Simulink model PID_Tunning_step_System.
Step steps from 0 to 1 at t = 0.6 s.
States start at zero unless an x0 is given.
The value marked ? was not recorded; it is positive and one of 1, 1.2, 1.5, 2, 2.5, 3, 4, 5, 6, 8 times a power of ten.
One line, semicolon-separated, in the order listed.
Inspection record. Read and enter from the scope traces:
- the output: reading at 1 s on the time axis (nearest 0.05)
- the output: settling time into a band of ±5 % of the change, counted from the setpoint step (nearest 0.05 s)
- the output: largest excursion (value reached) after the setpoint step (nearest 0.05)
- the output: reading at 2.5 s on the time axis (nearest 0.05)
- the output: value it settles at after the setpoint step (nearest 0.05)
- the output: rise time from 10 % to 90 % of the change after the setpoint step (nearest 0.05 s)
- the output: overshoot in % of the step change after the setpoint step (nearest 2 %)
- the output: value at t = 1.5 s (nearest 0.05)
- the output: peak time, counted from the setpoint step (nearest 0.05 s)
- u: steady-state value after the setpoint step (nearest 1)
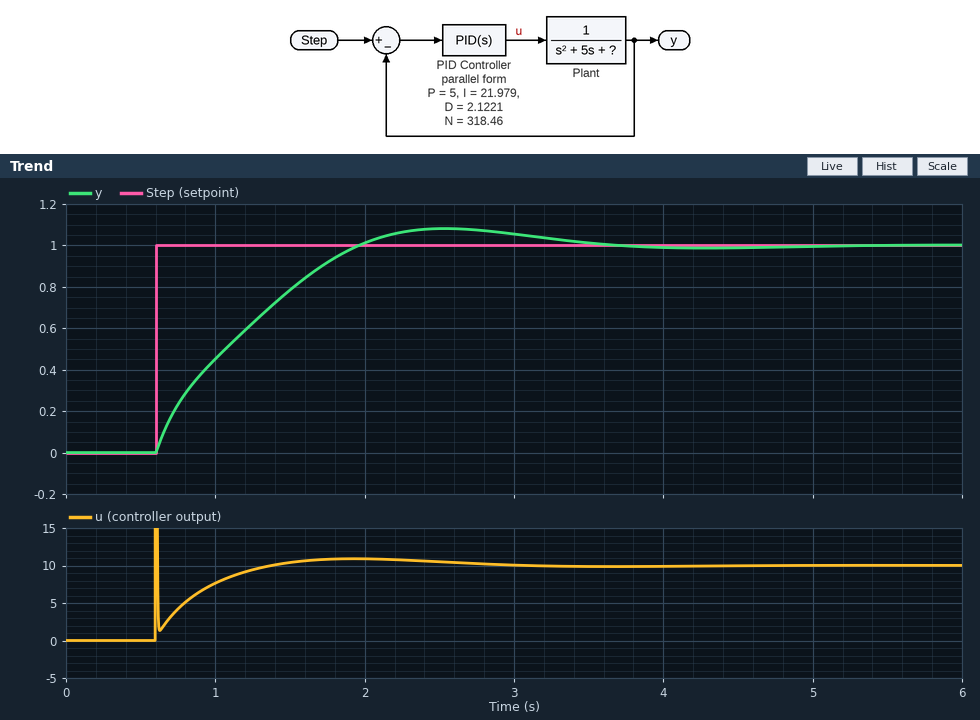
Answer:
0.45; 2.45 s; 1.10; 1.10; 1.00; 1.05 s; 8 %; 0.80; 1.95 s; 10
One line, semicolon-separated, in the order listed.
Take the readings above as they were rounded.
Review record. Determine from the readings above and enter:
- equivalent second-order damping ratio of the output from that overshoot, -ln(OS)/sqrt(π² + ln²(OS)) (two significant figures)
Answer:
0.63
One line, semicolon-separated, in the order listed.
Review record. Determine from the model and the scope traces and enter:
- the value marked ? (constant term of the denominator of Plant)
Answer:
10
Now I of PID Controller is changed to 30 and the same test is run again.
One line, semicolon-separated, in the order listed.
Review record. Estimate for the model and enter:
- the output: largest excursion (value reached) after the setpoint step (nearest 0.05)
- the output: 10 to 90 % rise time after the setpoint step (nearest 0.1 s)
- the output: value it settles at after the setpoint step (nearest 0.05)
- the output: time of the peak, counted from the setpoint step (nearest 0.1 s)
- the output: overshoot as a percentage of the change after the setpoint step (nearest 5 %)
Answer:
1.15; 0.8 s; 1.00; 1.6 s; 15 %
